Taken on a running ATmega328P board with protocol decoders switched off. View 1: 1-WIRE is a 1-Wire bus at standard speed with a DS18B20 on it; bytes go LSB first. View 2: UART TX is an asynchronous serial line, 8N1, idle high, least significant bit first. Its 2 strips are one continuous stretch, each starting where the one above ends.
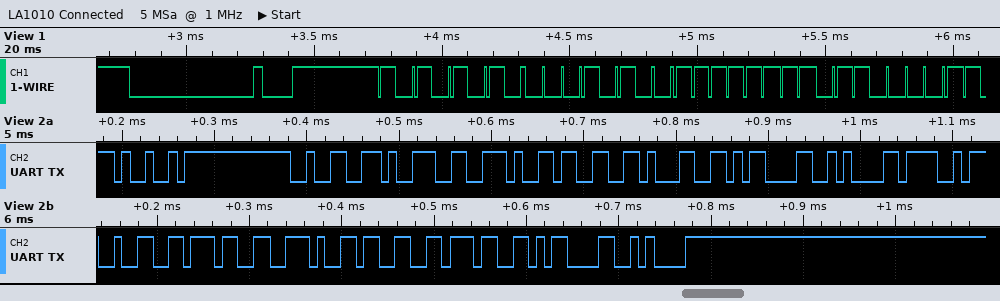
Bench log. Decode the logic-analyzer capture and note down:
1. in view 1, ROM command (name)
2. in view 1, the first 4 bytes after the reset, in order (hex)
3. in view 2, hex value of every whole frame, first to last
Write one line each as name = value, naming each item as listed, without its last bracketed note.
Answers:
in view 1, ROM command = Match ROM
in view 1, the first 4 bytes after the reset, in order = 55 28 FF 86
in view 2, hex value of every whole frame, first to last = 49 32 39 2E 33 31 0D 0A 4F 32 37 2E 33 37 0D 0A
